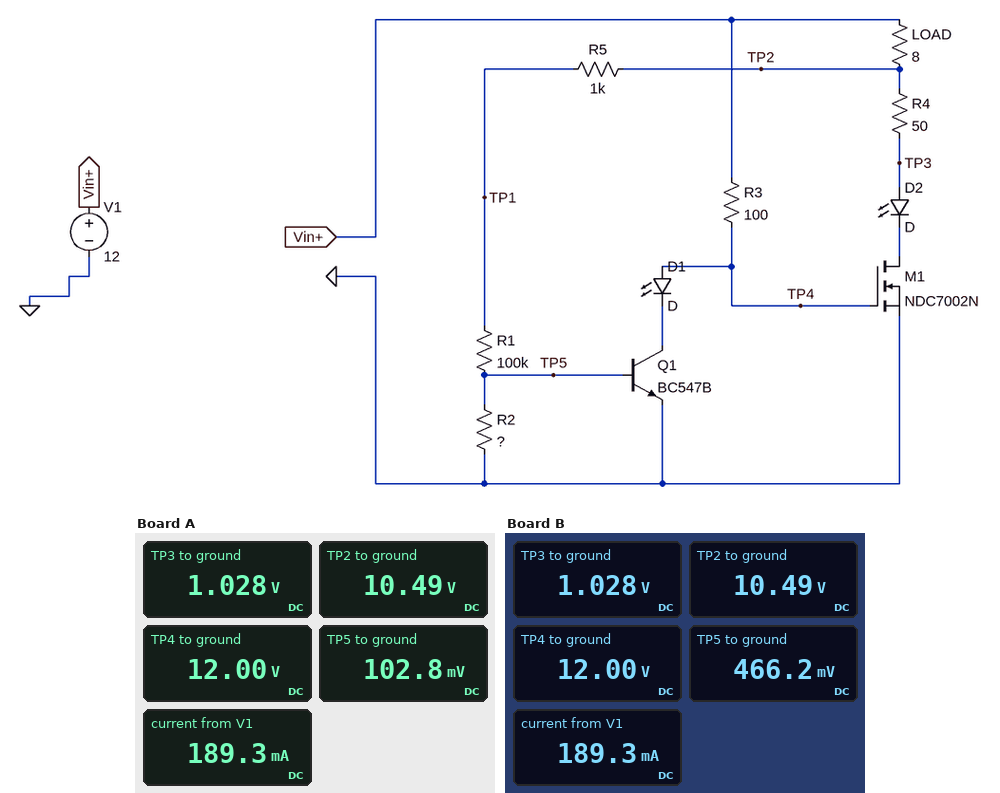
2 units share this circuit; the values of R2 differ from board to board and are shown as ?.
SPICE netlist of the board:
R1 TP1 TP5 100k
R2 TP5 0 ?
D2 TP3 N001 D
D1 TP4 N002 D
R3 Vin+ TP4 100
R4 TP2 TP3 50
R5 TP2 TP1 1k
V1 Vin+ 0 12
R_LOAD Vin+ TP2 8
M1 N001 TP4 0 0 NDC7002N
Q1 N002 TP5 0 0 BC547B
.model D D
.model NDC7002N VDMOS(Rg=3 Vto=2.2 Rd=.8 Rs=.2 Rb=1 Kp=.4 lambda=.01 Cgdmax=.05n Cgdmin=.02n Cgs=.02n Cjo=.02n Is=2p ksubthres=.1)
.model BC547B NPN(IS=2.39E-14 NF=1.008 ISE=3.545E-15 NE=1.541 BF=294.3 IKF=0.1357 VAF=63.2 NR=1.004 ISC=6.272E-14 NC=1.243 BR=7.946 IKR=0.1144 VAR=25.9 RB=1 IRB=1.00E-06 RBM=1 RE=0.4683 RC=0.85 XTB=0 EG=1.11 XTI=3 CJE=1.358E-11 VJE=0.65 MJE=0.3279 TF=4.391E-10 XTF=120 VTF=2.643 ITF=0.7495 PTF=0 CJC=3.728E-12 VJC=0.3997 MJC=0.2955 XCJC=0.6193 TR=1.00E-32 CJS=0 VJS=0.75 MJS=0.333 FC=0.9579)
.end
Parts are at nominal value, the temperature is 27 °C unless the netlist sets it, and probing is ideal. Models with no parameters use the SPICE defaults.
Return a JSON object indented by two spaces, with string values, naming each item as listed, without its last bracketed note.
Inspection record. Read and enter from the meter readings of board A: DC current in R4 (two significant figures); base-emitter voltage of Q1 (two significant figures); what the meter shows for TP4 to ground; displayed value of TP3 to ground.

{
  "DC current in R4": "190 mA",
  "base-emitter voltage of Q1": "100 mV",
  "what the meter shows for TP4 to ground": "12.00 V",
  "displayed value of TP3 to ground": "1.028 V"
}
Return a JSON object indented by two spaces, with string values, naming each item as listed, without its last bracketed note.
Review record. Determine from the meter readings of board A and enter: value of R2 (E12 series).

{
  "value of R2": "1 kΩ"
}
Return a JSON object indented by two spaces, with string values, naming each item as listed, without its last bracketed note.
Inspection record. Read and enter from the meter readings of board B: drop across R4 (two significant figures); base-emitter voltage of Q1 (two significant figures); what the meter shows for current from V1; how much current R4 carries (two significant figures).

{
  "drop across R4": "9.5 V",
  "base-emitter voltage of Q1": "470 mV",
  "what the meter shows for current from V1": "189.3 mA",
  "how much current R4 carries": "190 mA"
}
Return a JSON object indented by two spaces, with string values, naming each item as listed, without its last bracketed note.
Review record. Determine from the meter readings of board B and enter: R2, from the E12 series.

{
  "R2, from the E12 series": "4.7 kΩ"
}
